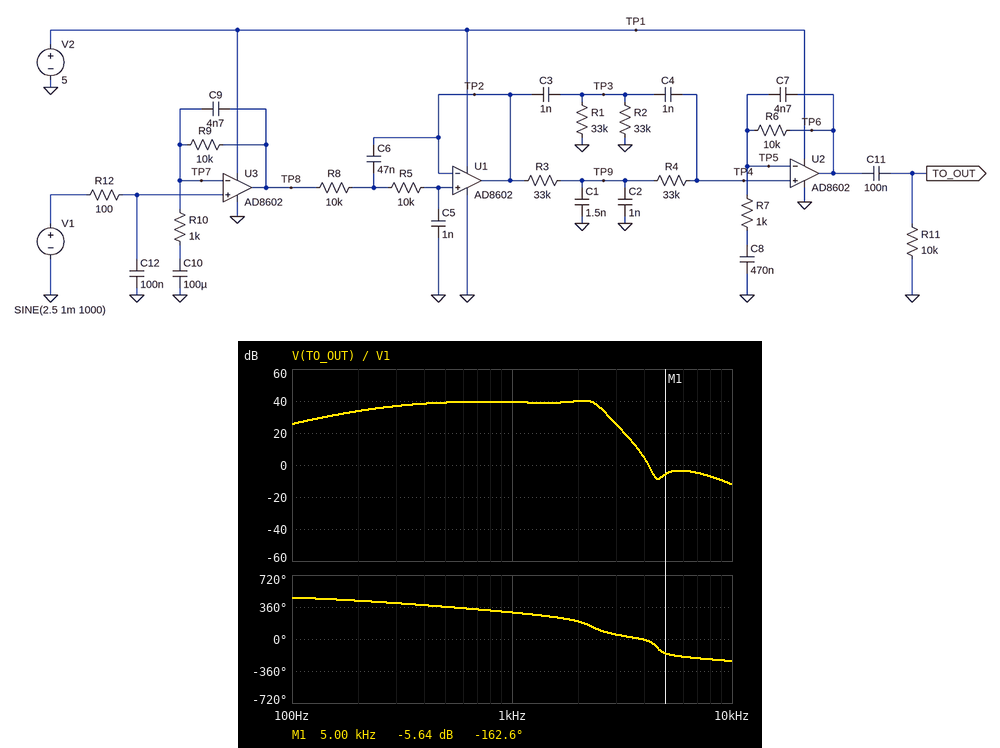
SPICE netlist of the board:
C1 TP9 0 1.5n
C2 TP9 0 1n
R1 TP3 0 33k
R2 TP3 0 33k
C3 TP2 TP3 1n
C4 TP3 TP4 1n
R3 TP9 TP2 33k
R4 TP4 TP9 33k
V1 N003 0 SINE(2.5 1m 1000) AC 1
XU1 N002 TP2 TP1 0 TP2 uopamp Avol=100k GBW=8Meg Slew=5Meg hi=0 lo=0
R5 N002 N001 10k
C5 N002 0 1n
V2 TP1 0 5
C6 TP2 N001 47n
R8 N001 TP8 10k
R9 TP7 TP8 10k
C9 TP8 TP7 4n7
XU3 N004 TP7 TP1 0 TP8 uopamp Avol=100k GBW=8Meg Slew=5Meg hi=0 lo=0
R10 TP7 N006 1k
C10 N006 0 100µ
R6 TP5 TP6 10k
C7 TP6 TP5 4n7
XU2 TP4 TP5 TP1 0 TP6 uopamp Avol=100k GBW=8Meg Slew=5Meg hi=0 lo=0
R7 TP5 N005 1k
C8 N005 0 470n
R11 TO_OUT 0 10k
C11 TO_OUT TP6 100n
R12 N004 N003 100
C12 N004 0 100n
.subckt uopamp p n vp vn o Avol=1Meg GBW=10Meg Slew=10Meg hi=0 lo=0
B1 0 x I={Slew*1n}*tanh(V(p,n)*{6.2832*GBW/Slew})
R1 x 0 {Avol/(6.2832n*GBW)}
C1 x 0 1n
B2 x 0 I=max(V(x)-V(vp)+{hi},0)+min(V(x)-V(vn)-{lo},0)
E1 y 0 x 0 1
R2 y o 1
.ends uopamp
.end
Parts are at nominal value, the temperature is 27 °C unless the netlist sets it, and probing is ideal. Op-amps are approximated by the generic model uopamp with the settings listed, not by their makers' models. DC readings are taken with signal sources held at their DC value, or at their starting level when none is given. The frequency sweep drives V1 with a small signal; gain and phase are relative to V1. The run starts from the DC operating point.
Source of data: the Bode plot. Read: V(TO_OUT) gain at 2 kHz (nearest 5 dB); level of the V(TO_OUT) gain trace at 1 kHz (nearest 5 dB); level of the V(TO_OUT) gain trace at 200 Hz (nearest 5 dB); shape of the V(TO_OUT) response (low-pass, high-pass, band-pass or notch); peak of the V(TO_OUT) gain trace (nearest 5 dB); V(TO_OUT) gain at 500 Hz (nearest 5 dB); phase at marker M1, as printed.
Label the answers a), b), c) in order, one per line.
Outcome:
a) 40 dB
b) 40 dB
c) 35 dB
d) band-pass
e) 40 dB
f) 40 dB
g) -162.6 deg
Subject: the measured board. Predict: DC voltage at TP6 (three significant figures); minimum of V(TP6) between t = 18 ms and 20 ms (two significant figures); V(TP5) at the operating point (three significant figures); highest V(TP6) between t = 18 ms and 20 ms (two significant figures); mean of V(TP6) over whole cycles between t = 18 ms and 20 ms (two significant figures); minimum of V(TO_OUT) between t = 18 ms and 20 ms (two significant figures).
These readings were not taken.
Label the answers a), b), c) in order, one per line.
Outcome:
a) 2.50 V
b) 2.4 V
c) 2.50 V
d) 2.6 V
e) 2.5 V
f) -92 mV
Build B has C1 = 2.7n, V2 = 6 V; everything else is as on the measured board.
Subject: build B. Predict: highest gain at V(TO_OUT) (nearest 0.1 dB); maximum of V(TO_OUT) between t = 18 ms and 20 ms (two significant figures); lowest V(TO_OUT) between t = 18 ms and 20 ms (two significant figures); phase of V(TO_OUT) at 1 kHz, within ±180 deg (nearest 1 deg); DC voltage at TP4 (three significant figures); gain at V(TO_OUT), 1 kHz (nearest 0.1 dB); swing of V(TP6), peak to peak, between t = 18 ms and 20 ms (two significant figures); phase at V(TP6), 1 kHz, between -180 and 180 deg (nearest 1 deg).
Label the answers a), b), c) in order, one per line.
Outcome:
a) 38.9 dB
b) 82 mV
c) -82 mV
d) -70 deg
e) 2.50 V
f) 38.3 dB
g) 170 mV
h) -79 deg
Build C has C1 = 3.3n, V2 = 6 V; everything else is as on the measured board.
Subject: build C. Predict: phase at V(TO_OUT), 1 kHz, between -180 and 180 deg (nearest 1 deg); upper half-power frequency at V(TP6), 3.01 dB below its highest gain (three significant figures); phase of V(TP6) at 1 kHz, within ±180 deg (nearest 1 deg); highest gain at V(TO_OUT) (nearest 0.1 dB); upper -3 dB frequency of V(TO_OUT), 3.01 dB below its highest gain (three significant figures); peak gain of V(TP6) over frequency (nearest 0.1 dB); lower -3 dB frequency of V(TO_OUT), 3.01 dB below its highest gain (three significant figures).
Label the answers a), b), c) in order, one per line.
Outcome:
a) -74 deg
b) 2.34 kHz
c) -83 deg
d) 38.6 dB
e) 2.36 kHz
f) 38.9 dB
g) 255 Hz
